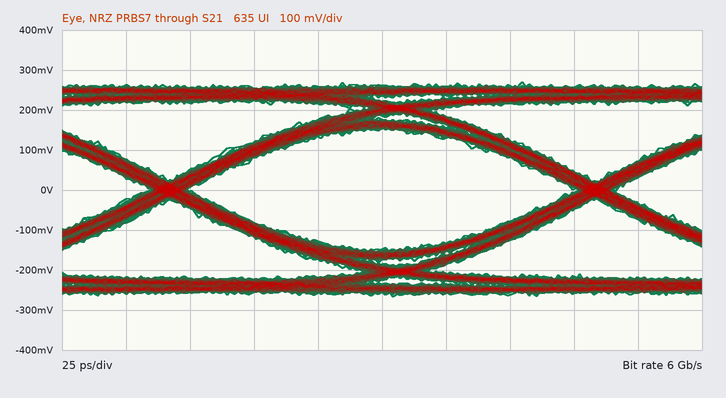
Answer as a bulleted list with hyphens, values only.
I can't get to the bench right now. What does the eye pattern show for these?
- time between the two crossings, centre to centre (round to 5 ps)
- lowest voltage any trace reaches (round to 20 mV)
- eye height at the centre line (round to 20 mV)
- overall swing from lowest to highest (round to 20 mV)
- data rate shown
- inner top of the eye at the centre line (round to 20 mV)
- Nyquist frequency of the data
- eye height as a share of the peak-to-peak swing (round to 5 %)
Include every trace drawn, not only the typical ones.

- 165 ps
- -260 mV
- 300 mV
- 540 mV
- 6 Gb/s
- 160 mV
- 3 GHz
- 55 %
